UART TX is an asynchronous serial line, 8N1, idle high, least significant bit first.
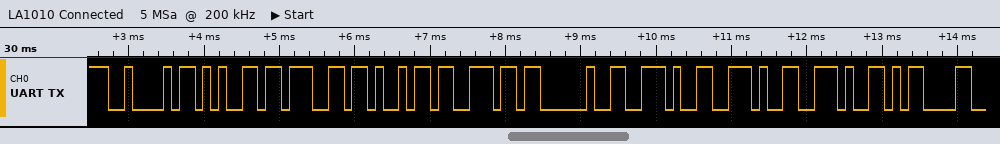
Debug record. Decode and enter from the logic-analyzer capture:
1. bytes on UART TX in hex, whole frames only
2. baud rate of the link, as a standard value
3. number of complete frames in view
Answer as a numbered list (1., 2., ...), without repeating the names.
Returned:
1. 0x42 0x65 0x67 0x69 0x6E 0x20 0x2E 0x2E 0x2E 0x0D
2. 9600 baud
3. 10
